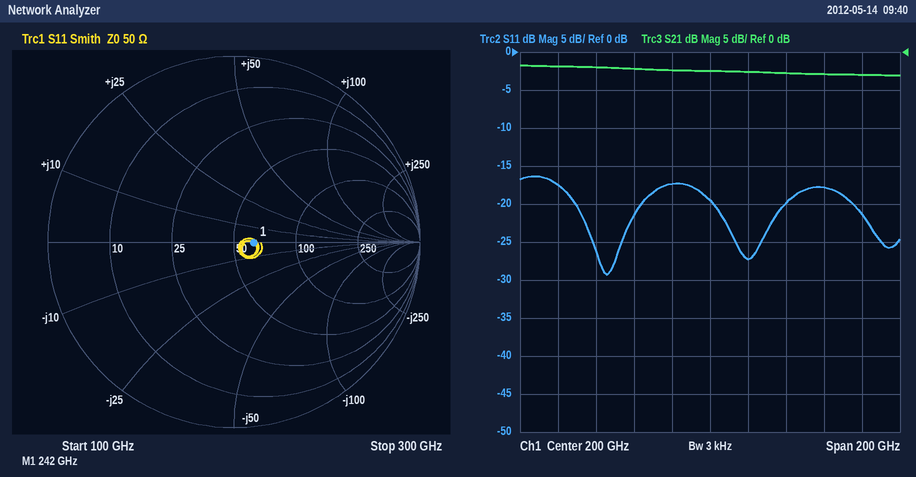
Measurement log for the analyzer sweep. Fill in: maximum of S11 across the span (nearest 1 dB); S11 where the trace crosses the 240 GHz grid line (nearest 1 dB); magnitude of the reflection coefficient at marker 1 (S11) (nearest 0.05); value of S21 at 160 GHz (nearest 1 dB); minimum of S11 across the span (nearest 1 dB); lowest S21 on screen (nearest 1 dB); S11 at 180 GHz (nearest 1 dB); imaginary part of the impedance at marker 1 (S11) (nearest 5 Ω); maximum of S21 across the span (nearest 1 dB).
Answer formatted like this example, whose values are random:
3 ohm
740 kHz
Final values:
-16 dB
-20 dB
0.10
-2 dB
-29 dB
-3 dB
-17 dB
0 Ω
-2 dB
